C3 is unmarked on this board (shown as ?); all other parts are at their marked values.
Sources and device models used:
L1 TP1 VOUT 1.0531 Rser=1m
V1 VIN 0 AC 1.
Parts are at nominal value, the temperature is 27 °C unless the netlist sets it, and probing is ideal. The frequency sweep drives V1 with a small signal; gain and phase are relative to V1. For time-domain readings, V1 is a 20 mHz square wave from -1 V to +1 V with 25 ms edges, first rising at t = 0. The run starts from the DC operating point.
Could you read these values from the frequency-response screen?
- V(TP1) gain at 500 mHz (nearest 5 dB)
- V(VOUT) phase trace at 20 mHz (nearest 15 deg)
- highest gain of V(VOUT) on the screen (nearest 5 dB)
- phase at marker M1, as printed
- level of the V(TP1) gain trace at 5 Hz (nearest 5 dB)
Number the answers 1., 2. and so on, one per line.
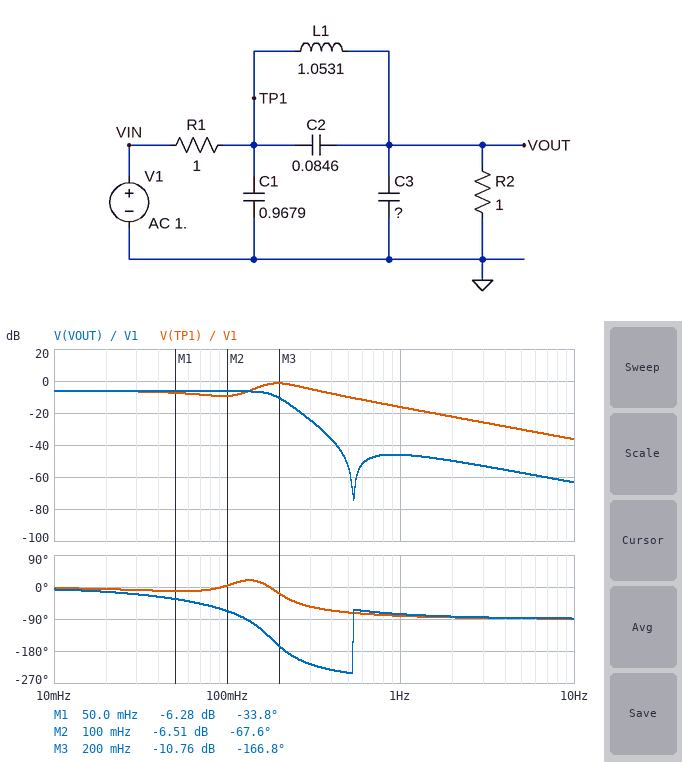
1. -10 dB
2. -15 deg
3. -5 dB
4. -33.8 deg
5. -30 dB
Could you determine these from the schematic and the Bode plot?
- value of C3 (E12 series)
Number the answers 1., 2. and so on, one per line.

1. 1.8 F
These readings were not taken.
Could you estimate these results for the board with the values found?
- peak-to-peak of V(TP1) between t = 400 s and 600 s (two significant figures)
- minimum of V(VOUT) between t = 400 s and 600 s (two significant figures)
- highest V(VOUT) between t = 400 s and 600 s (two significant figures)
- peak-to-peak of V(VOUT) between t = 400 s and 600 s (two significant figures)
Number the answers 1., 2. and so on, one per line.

1. 1.3 V
2. -590 mV
3. 590 mV
4. 1.2 V
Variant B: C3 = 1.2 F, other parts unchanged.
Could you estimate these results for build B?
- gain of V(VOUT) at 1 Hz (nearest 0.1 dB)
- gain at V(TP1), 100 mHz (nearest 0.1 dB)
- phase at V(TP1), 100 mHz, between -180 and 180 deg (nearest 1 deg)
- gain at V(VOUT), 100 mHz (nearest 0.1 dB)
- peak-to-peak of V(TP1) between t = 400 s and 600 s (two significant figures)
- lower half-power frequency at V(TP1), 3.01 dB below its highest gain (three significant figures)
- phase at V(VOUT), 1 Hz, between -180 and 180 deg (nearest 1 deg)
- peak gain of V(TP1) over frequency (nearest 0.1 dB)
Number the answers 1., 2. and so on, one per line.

1. -42.7 dB
2. -7.7 dB
3. -4 deg
4. -6.2 dB
5. 1.3 V
6. 151 mHz
7. -74 deg
8. -2.2 dB
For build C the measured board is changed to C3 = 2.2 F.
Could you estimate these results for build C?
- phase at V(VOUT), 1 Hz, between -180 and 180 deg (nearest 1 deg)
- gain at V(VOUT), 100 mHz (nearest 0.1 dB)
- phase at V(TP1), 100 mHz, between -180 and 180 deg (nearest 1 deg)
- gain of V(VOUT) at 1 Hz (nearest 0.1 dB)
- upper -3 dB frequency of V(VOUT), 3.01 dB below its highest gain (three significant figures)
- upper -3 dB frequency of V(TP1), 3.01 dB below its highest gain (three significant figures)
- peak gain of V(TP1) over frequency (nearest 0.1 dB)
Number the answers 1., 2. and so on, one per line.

1. -77 deg
2. -6.8 dB
3. 12 deg
4. -47.8 dB
5. 173 mHz
6. 277 mHz
7. -1.1 dB
